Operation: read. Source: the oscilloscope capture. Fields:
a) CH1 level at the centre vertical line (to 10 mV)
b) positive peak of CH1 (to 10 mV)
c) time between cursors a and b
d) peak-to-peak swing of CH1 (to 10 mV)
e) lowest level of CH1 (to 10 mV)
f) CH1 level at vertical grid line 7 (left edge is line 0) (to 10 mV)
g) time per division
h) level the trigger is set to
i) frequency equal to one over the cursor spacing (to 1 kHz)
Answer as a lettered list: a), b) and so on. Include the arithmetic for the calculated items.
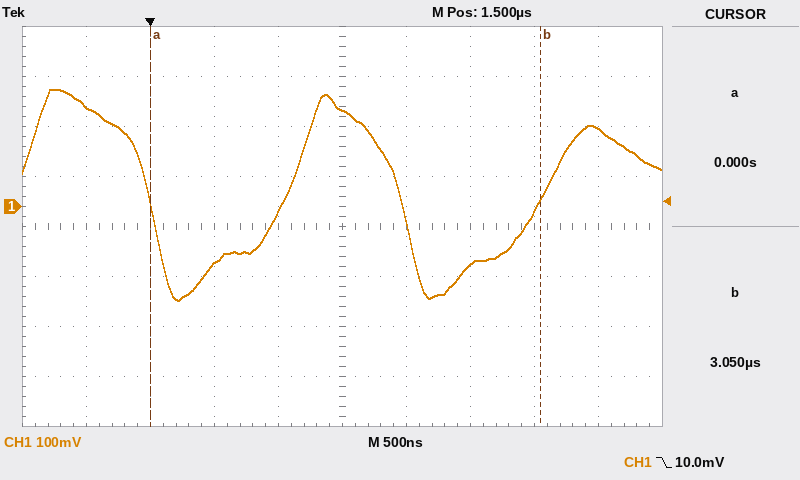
a) 190 mV
b) 230 mV
c) 3.05 µs − (0 s) = 3.05 µs
d) 230 mV − (-190 mV) = 420 mV
e) -190 mV
f) -120 mV
g) 500 ns
h) 10.0 mV
i) 1 / 3.05 µs ≈ 328 kHz
